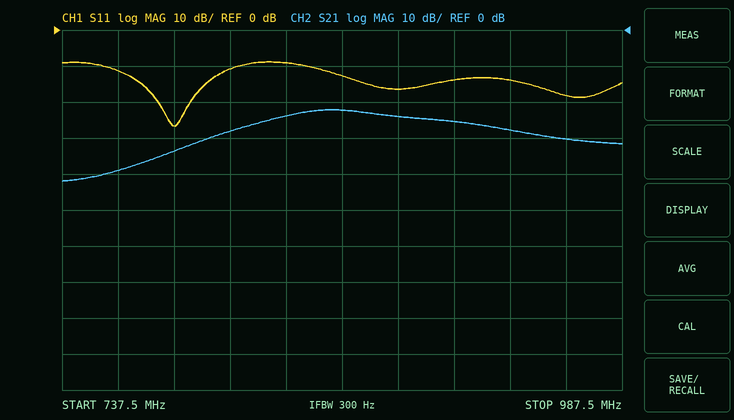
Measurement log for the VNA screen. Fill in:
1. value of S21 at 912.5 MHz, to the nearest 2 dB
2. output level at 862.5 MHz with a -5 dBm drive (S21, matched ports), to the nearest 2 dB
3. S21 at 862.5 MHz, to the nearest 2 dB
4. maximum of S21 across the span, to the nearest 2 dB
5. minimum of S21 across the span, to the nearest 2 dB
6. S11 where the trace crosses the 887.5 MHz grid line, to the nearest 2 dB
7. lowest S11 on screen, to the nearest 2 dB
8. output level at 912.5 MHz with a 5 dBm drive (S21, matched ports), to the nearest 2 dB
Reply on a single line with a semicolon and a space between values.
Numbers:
-26 dB; -28 dBm; -22 dB; -22 dB; -42 dB; -16 dB; -26 dB; -20 dBm
